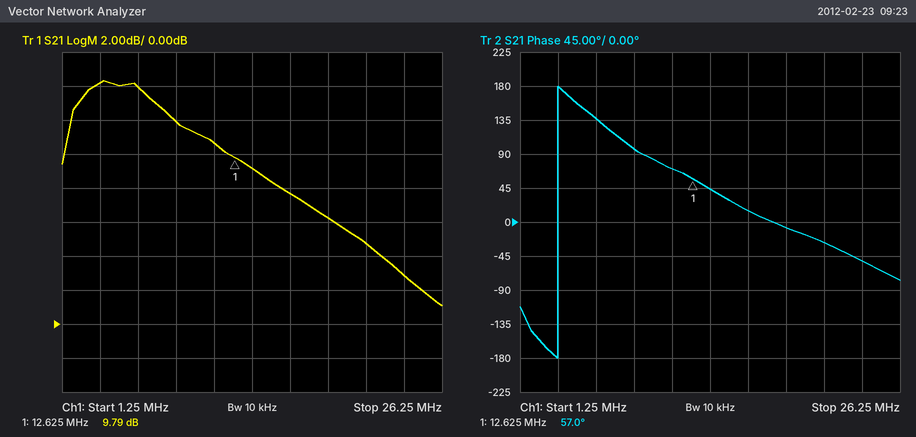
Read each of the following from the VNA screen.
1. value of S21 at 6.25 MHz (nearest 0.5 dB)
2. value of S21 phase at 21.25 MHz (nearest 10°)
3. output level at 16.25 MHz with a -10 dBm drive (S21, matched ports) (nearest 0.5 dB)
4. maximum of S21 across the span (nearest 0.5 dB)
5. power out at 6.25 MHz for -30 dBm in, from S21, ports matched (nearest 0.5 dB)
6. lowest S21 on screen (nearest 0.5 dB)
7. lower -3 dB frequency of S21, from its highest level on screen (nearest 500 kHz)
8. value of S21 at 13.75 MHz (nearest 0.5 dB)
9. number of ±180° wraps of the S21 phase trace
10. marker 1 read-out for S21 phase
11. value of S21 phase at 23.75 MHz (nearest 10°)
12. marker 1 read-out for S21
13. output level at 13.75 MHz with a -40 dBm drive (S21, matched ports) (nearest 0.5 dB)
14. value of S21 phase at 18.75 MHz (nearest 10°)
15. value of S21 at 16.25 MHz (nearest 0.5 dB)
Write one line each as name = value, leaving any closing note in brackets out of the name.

value of S21 at 6.25 MHz = 14.0 dB
value of S21 phase at 21.25 MHz = -30°
output level at 16.25 MHz with a -10 dBm drive (S21, matched ports) = -2.5 dBm
maximum of S21 across the span = 14.5 dB
power out at 6.25 MHz for -30 dBm in, from S21, ports matched = -16.0 dBm
lowest S21 on screen = 1.0 dB
lower -3 dB frequency of S21, from its highest level on screen = 1.5 MHz
value of S21 at 13.75 MHz = 9.0 dB
number of ±180° wraps of the S21 phase trace = 1
marker 1 read-out for S21 phase = 57.0°
value of S21 phase at 23.75 MHz = -50°
marker 1 read-out for S21 = 9.79 dB
output level at 13.75 MHz with a -40 dBm drive (S21, matched ports) = -31.0 dBm
value of S21 phase at 18.75 MHz = -10°
value of S21 at 16.25 MHz = 7.5 dB
